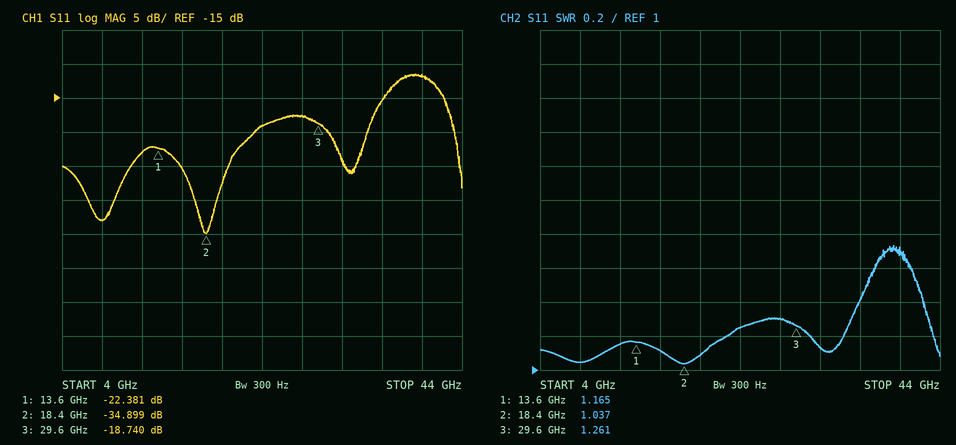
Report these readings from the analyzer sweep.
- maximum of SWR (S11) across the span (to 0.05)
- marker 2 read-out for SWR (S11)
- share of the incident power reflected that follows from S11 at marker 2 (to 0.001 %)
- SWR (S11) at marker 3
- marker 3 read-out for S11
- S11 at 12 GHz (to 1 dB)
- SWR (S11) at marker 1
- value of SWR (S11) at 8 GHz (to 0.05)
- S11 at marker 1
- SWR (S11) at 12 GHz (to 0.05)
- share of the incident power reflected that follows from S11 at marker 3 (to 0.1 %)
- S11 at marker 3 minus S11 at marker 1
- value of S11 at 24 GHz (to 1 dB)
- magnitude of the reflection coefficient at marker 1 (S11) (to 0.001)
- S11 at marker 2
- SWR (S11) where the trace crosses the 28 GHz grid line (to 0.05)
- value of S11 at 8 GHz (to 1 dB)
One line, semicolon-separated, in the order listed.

1.75; 1.037; 0.032 %; 1.261; -18.740 dB; -23 dB; 1.165; 1.05; -22.381 dB; 1.15; 1.3 %; 3.641 dB; -19 dB; 0.076; -34.899 dB; 1.30; -33 dB
